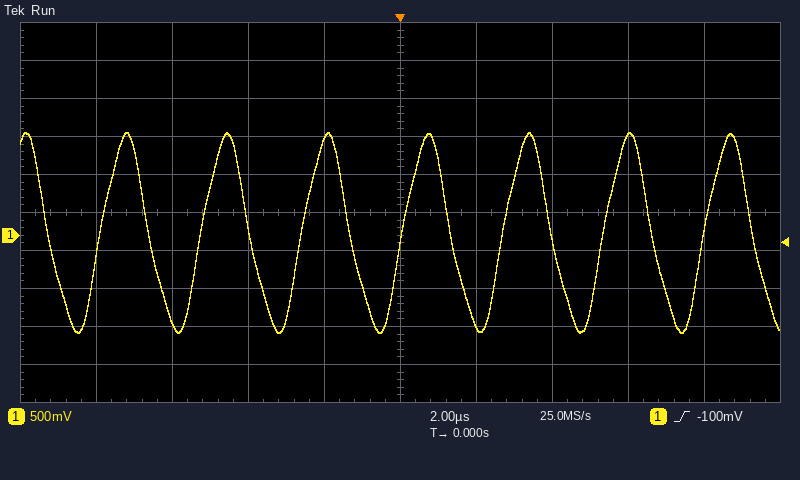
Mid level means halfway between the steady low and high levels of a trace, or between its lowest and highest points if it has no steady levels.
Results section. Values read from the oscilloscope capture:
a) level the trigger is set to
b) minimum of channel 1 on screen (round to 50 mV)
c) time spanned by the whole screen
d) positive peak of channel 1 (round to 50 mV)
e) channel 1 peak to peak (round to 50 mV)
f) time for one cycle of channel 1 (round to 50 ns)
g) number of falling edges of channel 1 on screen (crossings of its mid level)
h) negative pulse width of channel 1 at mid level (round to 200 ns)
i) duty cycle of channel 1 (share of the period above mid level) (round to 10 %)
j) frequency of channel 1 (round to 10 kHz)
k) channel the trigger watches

-100 mV
-1.30 V
20 µs
1.35 V
2.65 V
2.65 µs
8
1.4 µs
50 %
380 kHz
channel 1
